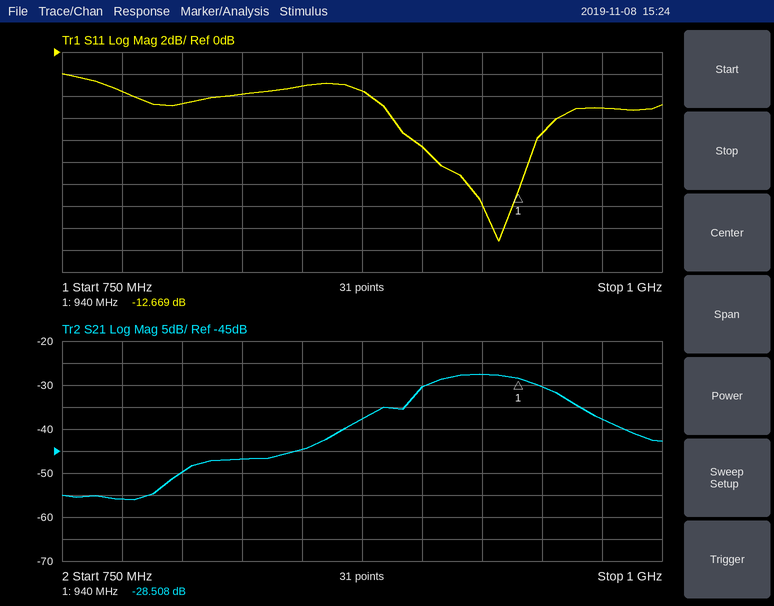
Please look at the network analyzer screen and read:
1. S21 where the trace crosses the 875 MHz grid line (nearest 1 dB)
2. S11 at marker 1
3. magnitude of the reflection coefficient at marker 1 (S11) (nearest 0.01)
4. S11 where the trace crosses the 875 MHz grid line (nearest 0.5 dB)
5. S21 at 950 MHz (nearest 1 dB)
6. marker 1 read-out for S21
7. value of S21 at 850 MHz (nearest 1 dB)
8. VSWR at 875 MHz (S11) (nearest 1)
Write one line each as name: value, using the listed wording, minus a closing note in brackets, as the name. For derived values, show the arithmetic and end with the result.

S21 where the trace crosses the 875 MHz grid line: -38 dB
S11 at marker 1: -12.669 dB
magnitude of the reflection coefficient at marker 1 (S11): 10^(-12.669/20) ≈ 0.23
S11 where the trace crosses the 875 MHz grid line: -3.5 dB
S21 at 950 MHz: -30 dB
marker 1 read-out for S21: -28.508 dB
value of S21 at 850 MHz: -45 dB
VSWR at 875 MHz (S11): |Γ| = 10^(-3.5/20) = 0.6683; VSWR = (1 + 0.6683)/(1 − 0.6683) ≈ 5
